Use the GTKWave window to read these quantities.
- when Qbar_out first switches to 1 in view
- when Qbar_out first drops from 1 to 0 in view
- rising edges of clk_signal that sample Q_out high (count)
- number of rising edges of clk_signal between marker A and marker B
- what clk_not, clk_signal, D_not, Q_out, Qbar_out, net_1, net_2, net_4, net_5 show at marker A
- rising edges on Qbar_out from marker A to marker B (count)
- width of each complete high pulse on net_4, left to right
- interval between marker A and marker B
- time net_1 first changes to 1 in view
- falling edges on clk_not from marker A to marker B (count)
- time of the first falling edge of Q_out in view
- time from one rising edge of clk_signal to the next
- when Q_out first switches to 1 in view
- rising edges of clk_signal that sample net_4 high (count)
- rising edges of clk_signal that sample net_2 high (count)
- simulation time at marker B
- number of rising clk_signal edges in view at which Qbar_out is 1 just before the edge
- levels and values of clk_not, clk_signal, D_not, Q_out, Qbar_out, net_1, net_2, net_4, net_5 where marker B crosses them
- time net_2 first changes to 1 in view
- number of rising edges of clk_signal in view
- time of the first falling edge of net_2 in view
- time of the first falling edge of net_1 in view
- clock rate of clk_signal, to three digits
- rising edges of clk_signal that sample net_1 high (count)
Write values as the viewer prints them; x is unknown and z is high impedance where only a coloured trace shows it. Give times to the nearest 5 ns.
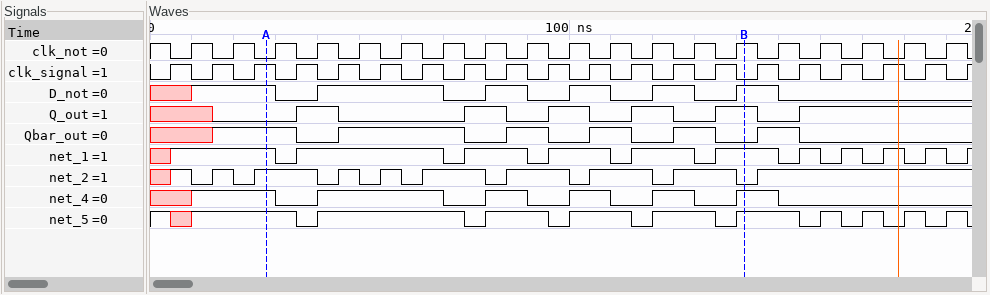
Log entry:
15 ns
35 ns
9
11
clk_not=0, clk_signal=1, D_not=1, Q_out=0, Qbar_out=1, net_1=1, net_2=1, net_4=1, net_5=1
4
30 ns, 10 ns, 10 ns, 10 ns, 10 ns
115 ns
5 ns
11
45 ns
10 ns
35 ns
9
10
140 ns
9
clk_not=1, clk_signal=0, D_not=1, Q_out=1, Qbar_out=0, net_1=1, net_2=0, net_4=1, net_5=1
5 ns
20
10 ns
30 ns
100 MHz
9
